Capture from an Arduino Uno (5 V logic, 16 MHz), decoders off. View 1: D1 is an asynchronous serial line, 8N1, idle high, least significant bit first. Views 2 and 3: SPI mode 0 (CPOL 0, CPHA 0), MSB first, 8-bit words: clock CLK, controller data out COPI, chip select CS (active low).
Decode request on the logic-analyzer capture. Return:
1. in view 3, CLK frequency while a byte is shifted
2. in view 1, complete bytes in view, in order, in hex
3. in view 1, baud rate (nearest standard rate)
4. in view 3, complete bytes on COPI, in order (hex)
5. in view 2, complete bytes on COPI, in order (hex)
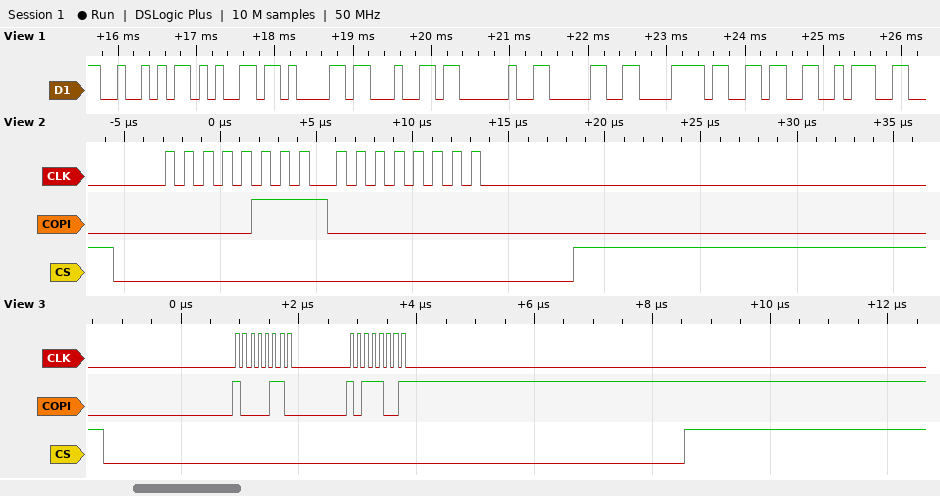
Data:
8 MHz
52 65 61 64 20 30 78 36 3A
9600 baud
86 B9
07 00
